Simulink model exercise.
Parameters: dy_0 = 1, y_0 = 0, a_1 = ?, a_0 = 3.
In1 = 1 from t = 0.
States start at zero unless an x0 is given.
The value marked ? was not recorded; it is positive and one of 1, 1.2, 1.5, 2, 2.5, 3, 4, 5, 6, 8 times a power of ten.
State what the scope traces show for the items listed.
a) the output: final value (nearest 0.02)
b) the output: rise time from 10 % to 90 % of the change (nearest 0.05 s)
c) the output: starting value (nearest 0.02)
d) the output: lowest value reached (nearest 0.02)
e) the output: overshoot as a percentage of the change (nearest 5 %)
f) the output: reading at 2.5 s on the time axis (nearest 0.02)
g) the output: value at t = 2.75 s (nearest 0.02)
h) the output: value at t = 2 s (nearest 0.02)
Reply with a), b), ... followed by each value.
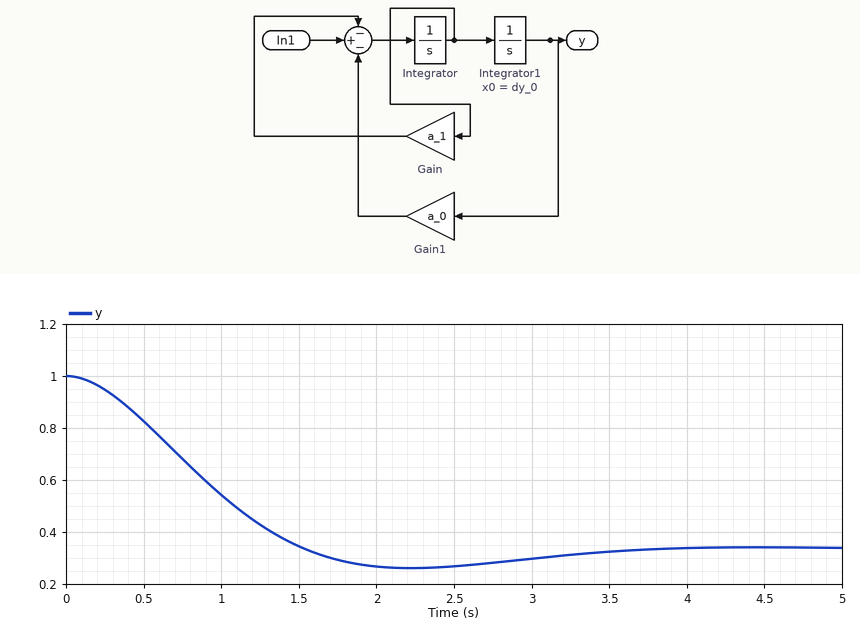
a) 0.34
b) 1.05 s
c) 1.00
d) 0.26
e) 10 %
f) 0.26
g) 0.28
h) 0.26
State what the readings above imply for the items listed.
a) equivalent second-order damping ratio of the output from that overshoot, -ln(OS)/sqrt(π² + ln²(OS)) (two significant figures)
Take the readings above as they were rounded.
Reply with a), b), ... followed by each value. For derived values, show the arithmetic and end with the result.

a) ln(0.1) = -2.303; 2.303 / sqrt(9.870 + 5.302) = 0.59
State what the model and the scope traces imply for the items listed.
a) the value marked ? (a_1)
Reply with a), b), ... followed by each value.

a) 2
